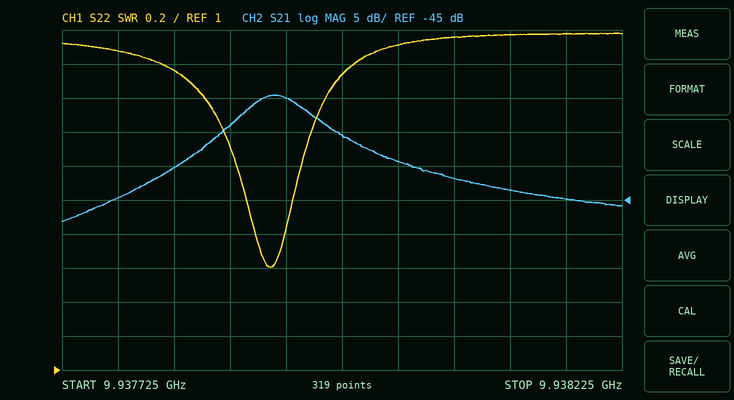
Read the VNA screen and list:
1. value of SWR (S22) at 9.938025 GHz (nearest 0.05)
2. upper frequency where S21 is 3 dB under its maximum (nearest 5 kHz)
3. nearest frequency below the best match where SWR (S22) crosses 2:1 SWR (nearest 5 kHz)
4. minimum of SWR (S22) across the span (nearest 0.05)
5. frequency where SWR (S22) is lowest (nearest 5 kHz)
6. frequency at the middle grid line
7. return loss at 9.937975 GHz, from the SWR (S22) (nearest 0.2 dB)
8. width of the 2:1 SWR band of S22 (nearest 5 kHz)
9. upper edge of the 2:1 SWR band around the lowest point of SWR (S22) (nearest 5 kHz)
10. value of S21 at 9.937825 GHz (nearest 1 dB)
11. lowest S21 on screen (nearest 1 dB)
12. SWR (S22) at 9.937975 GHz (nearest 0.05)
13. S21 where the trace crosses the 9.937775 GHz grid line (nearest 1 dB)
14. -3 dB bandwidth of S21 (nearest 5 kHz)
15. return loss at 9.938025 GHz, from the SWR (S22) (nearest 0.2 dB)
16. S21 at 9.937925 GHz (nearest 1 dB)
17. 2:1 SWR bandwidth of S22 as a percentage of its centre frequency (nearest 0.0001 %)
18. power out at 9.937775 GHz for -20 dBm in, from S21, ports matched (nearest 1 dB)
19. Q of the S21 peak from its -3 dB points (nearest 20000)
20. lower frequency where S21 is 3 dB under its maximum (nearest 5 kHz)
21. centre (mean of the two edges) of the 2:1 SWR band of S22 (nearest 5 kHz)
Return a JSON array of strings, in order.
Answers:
["2.90", "9.937950 GHz", "9.937890 GHz", "1.60", "9.937910 GHz", "9.937975 GHz", "6.6 dB", "40 kHz", "9.937930 GHz", "-40 dB", "-48 dB", "2.75", "-45 dB", "65 kHz", "6.2 dB", "-30 dB", "0.0004 %", "-65 dBm", "160000", "9.937885 GHz", "9.937910 GHz"]
